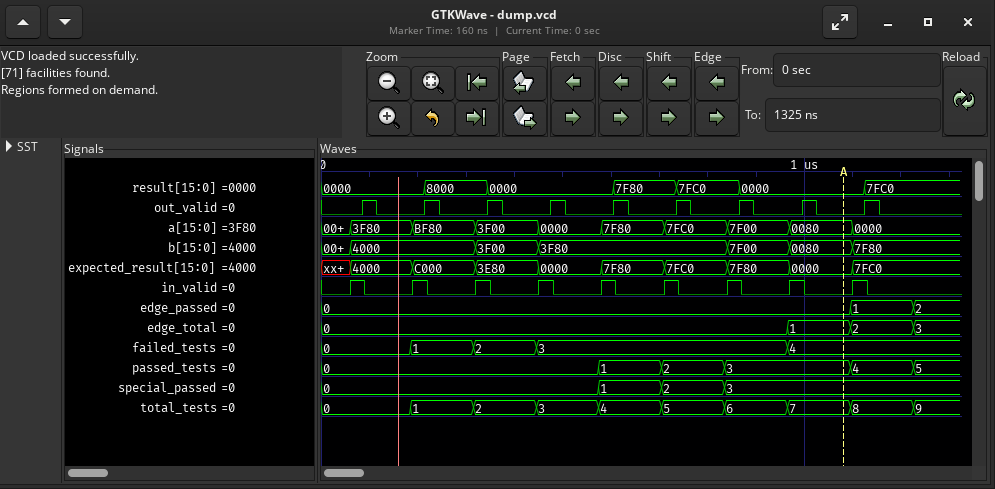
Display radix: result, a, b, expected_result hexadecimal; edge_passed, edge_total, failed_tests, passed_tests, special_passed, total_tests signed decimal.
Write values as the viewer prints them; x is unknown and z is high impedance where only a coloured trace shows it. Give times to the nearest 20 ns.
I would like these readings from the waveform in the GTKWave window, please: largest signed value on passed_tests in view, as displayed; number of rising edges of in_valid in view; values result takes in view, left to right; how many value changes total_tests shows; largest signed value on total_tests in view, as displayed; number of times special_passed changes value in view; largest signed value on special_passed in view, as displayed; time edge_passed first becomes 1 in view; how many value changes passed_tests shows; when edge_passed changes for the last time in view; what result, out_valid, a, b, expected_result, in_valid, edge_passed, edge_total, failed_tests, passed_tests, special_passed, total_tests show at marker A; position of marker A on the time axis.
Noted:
5
9
0000, 8000, 0000, 7F80, 7FC0, 0000, 7FC0
9
9
3
3
1100 ns
5
1220 ns
result=0000, out_valid=0, a=0080, b=0080, expected_result=0000, in_valid=0, edge_passed=0, edge_total=1, failed_tests=4, passed_tests=3, special_passed=3, total_tests=7
1080 ns
